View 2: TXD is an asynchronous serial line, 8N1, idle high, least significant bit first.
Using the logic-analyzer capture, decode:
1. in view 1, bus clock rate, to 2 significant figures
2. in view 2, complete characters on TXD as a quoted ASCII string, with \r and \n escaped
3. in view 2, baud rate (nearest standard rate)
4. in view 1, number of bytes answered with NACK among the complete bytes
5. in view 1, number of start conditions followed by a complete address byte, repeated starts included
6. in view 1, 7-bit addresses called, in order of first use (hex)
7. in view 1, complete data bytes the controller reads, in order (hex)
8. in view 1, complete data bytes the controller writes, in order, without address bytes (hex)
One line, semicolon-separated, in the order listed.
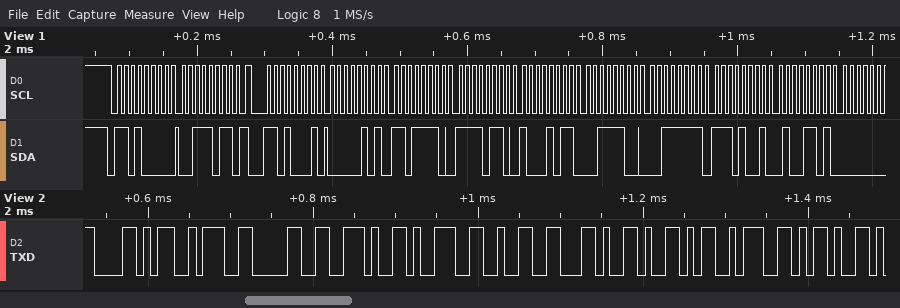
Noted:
100 kHz; "X:0.92,Y:-"; 115200 baud; 0; 2; 0x68; 05 DE F6 8B 3C 3F E9 4D; 3B
